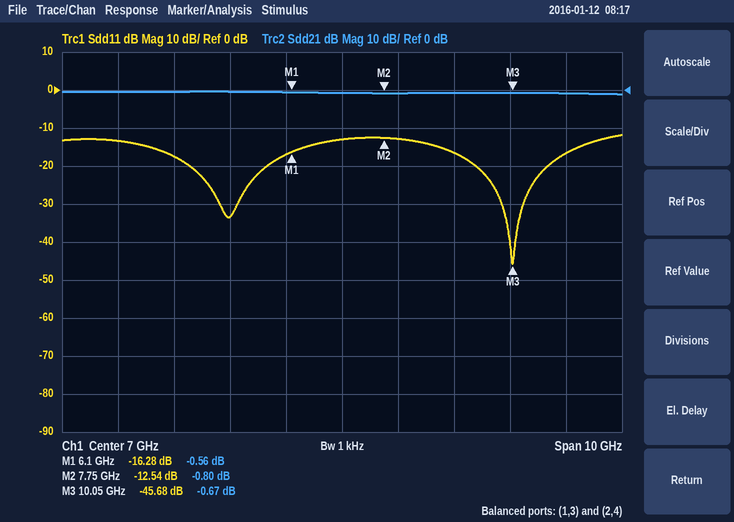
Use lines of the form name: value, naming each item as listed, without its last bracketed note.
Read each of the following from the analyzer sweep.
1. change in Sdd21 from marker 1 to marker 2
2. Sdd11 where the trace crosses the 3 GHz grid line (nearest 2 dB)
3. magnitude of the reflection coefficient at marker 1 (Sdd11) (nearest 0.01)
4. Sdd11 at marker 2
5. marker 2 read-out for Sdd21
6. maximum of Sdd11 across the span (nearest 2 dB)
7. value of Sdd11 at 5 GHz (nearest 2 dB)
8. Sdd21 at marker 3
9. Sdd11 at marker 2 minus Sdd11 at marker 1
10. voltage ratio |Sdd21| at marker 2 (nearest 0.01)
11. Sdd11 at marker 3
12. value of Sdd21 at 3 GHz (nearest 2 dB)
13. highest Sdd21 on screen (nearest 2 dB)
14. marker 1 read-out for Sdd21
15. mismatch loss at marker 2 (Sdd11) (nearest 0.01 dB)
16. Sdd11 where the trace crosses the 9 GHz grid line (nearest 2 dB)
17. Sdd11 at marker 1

change in Sdd21 from marker 1 to marker 2: -0.24 dB
Sdd11 where the trace crosses the 3 GHz grid line: -14 dB
magnitude of the reflection coefficient at marker 1 (Sdd11): 0.15
Sdd11 at marker 2: -12.54 dB
marker 2 read-out for Sdd21: -0.80 dB
maximum of Sdd11 across the span: -12 dB
value of Sdd11 at 5 GHz: -34 dB
Sdd21 at marker 3: -0.67 dB
Sdd11 at marker 2 minus Sdd11 at marker 1: 3.74 dB
voltage ratio |Sdd21| at marker 2: 0.91
Sdd11 at marker 3: -45.68 dB
value of Sdd21 at 3 GHz: 0 dB
highest Sdd21 on screen: 0 dB
marker 1 read-out for Sdd21: -0.56 dB
mismatch loss at marker 2 (Sdd11): 0.25 dB
Sdd11 where the trace crosses the 9 GHz grid line: -16 dB
Sdd11 at marker 1: -16.28 dB
